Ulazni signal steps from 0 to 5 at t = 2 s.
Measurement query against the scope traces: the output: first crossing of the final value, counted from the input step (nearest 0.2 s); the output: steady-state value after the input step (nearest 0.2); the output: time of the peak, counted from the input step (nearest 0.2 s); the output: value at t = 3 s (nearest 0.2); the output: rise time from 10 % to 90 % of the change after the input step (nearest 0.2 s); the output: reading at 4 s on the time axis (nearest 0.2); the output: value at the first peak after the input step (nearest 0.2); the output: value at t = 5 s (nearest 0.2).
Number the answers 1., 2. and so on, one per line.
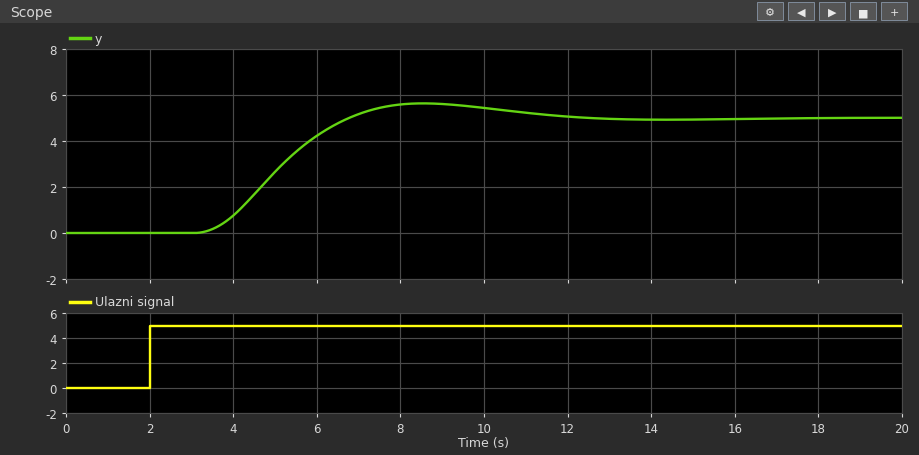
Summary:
1. 4.8 s
2. 5.0
3. 6.6 s
4. 0.0
5. 2.4 s
6. 0.8
7. 5.6
8. 2.6
